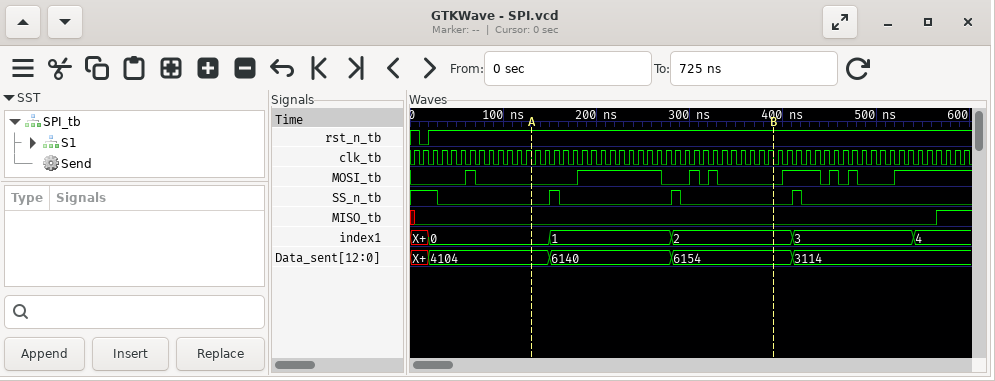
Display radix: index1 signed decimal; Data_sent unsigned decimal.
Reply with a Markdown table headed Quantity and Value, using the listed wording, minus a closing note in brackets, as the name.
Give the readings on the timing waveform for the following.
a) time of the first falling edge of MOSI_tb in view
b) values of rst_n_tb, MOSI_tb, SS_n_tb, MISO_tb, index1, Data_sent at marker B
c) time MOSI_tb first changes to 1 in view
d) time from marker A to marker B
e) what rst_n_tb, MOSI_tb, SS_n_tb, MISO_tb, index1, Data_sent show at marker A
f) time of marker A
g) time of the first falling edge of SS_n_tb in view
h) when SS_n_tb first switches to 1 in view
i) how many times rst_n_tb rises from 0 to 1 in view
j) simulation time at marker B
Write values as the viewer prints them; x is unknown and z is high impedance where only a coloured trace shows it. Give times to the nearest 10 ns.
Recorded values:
| Quantity | Value |
|---|---|
| time of the first falling edge of MOSI_tb in view | 70 ns |
| values of rst_n_tb, MOSI_tb, SS_n_tb, MISO_tb, index1, Data_sent at marker B | rst_n_tb=1, MOSI_tb=0, SS_n_tb=0, MISO_tb=0, index1=2, Data_sent=6154 |
| time MOSI_tb first changes to 1 in view | 60 ns |
| time from marker A to marker B | 260 ns |
| what rst_n_tb, MOSI_tb, SS_n_tb, MISO_tb, index1, Data_sent show at marker A | rst_n_tb=1, MOSI_tb=0, SS_n_tb=0, MISO_tb=0, index1=0, Data_sent=4104 |
| time of marker A | 130 ns |
| time of the first falling edge of SS_n_tb in view | 30 ns |
| when SS_n_tb first switches to 1 in view | 150 ns |
| how many times rst_n_tb rises from 0 to 1 in view | 1 |
| simulation time at marker B | 390 ns |
